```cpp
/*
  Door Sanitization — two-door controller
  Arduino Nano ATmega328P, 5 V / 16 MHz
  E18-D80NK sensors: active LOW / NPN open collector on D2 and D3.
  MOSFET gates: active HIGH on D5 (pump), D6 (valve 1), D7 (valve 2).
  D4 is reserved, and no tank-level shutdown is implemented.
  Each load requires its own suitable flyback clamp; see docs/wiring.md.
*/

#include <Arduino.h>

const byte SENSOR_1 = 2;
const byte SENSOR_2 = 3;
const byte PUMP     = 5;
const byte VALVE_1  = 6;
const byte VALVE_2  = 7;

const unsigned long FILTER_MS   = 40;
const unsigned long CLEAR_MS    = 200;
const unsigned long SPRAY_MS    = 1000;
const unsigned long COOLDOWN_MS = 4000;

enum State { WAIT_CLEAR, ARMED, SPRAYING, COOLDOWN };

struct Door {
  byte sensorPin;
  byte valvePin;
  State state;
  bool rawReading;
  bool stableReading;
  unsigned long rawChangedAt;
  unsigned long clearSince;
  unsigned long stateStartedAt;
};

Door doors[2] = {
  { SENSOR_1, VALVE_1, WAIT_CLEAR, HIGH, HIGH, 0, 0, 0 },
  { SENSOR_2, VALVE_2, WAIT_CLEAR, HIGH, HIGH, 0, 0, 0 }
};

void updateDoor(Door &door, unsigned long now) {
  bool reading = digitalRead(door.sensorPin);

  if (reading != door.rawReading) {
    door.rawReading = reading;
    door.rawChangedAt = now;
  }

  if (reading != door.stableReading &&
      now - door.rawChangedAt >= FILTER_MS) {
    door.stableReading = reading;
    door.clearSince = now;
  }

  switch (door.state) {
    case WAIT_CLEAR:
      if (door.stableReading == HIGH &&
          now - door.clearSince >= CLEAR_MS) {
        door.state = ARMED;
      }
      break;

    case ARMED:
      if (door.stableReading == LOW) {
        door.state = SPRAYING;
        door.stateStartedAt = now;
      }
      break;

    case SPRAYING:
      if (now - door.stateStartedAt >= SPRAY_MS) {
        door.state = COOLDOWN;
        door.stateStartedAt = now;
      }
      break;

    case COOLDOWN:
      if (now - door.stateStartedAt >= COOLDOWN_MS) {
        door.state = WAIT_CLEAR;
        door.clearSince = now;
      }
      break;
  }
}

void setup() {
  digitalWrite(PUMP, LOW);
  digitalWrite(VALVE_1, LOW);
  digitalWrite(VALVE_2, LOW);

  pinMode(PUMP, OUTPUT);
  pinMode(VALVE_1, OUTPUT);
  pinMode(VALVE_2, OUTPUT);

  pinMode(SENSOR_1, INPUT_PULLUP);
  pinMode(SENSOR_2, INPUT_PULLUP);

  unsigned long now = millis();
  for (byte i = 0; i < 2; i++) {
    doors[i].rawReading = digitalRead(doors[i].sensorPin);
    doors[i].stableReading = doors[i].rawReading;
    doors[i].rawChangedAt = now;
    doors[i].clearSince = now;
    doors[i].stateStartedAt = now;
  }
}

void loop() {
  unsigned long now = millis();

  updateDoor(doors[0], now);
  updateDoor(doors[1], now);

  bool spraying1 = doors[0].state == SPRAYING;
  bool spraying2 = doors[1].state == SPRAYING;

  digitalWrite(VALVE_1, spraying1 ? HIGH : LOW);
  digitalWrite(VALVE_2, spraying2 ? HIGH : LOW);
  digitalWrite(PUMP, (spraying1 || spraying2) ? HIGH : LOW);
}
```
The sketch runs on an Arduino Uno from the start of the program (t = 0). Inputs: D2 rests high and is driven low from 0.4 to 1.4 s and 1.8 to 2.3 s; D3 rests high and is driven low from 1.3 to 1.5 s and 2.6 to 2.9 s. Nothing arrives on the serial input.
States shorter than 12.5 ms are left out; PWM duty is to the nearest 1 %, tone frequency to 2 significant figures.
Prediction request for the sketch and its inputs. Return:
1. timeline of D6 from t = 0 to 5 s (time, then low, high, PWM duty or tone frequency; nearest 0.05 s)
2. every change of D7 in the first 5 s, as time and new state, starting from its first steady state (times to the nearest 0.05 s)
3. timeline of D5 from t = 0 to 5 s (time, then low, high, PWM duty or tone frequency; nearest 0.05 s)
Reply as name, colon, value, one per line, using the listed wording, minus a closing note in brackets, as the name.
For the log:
timeline of D6 from t = 0 to 5 s: 0 s low; 0.45 s high; 1.45 s low
every change of D7 in the first 5 s, as time and new state, starting from its first steady state: 0 s low; 1.35 s high; 2.35 s low
timeline of D5 from t = 0 to 5 s: 0 s low; 0.45 s high; 2.35 s low
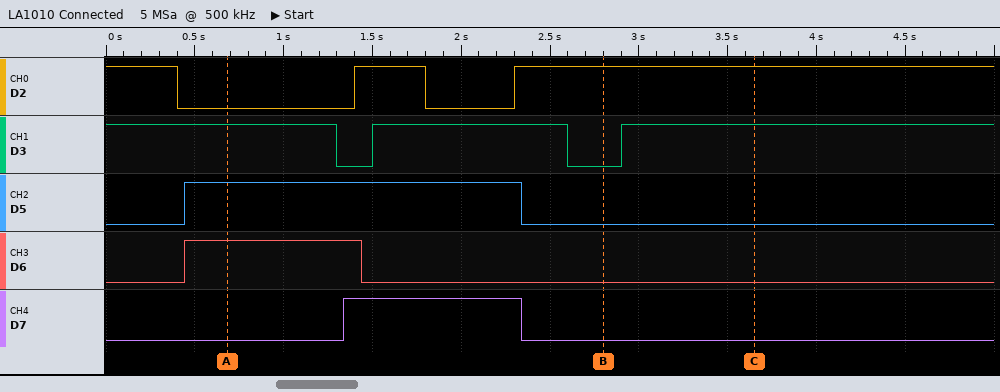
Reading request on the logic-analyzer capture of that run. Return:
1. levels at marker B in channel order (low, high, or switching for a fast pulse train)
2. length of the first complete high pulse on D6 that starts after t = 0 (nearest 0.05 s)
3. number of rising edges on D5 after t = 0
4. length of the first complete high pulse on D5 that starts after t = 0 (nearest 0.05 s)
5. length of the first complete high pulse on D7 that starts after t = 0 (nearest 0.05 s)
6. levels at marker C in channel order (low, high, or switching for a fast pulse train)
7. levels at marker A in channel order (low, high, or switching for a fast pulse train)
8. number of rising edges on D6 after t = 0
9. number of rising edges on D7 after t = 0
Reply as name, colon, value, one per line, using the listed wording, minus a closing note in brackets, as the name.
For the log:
levels at marker B in channel order: D2 high, D3 low, D5 low, D6 low, D7 low
length of the first complete high pulse on D6 that starts after t = 0: 1.00 s
number of rising edges on D5 after t = 0: 1
length of the first complete high pulse on D5 that starts after t = 0: 1.90 s
length of the first complete high pulse on D7 that starts after t = 0: 1.00 s
levels at marker C in channel order: D2 high, D3 high, D5 low, D6 low, D7 low
levels at marker A in channel order: D2 low, D3 high, D5 high, D6 high, D7 low
number of rising edges on D6 after t = 0: 1
number of rising edges on D7 after t = 0: 1
